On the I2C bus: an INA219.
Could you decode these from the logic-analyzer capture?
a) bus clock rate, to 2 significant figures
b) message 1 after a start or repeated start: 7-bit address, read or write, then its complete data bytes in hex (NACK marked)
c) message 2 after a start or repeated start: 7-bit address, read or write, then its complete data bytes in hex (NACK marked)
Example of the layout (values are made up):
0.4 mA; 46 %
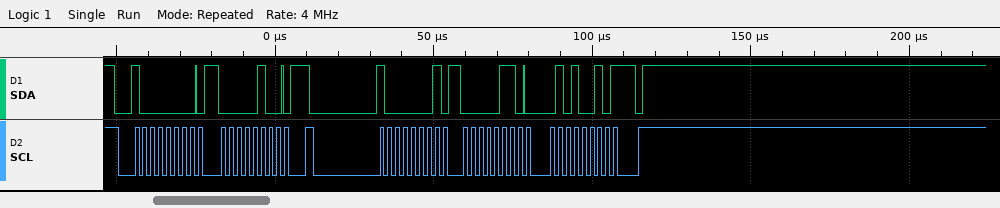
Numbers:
400 kHz; 0x40 write: 04; 0x40 read: 06 52 NACK
